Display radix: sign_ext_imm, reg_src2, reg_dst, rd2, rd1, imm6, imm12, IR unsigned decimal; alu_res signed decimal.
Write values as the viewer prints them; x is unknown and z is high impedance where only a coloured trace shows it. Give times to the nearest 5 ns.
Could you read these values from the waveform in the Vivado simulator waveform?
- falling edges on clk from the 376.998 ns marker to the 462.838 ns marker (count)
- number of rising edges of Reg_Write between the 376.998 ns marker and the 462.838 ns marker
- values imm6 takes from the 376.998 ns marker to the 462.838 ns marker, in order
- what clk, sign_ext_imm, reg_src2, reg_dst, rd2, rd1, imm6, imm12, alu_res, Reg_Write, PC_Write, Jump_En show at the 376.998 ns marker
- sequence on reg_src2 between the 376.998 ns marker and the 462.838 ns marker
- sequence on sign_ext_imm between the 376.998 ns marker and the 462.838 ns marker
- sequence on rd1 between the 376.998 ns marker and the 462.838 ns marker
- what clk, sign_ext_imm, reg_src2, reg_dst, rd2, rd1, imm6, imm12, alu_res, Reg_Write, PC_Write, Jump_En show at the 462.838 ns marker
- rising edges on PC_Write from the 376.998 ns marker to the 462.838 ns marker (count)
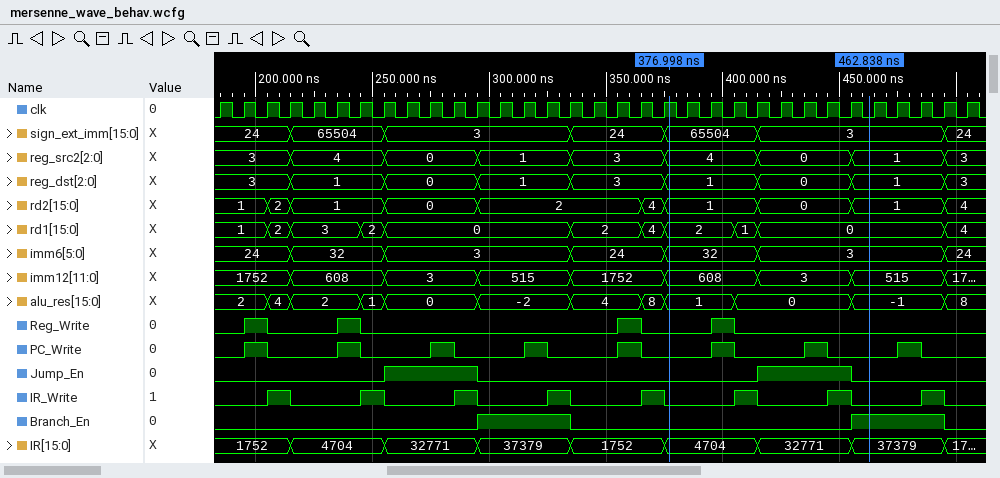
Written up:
9
1
32, 3
clk=1, sign_ext_imm=65504, reg_src2=4, reg_dst=1, rd2=1, rd1=2, imm6=32, imm12=608, alu_res=1, Reg_Write=0, PC_Write=0, Jump_En=0
4, 0, 1
65504, 3
2, 1, 0
clk=0, sign_ext_imm=3, reg_src2=1, reg_dst=1, rd2=1, rd1=0, imm6=3, imm12=515, alu_res=-1, Reg_Write=0, PC_Write=0, Jump_En=0
2
